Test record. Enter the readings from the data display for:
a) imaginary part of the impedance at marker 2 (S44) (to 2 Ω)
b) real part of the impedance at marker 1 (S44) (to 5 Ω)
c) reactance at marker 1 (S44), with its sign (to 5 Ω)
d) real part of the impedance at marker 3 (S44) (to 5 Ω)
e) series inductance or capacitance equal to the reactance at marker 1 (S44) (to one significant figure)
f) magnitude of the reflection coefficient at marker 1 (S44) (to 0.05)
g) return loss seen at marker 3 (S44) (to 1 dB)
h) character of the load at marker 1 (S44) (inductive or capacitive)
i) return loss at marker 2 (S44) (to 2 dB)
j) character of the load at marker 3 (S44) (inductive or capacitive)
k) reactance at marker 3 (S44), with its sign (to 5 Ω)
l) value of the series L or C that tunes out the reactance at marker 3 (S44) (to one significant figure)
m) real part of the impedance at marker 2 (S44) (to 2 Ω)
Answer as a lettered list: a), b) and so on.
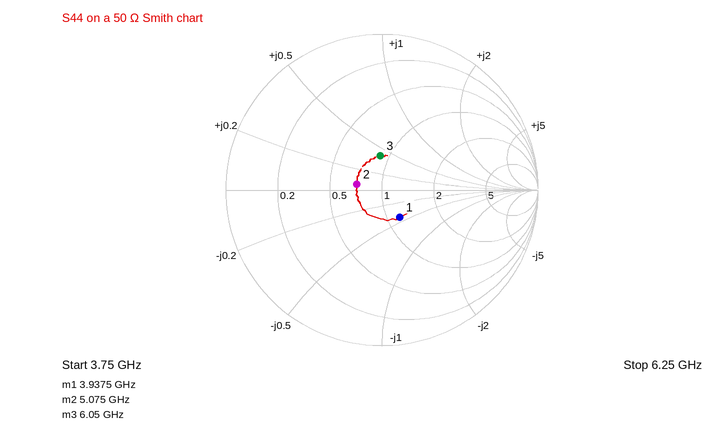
a) +2 Ω
b) 60 Ω
c) -20 Ω
d) 45 Ω
e) 2 pF
f) 0.20
g) 13 dB
h) capacitive
i) 16 dB
j) inductive
k) +20 Ω
l) 1 pF
m) 36 Ω
